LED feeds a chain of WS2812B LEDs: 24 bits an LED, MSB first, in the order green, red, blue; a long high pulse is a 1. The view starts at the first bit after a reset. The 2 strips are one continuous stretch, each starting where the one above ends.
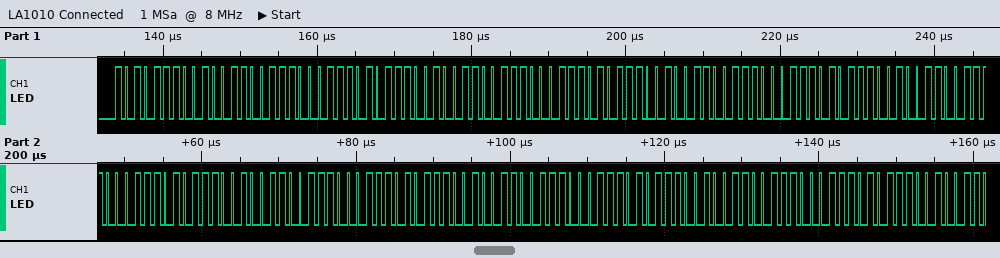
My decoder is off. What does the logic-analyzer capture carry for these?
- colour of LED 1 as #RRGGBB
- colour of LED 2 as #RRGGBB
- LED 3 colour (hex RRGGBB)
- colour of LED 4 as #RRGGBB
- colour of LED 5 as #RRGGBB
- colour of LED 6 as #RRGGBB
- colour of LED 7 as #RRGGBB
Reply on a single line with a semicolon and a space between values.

#4CAEE3; #4CAEE3; #4CAEE3; #4CAEE3; #4CAEE3; #4CAEE3; #4CAEE3
